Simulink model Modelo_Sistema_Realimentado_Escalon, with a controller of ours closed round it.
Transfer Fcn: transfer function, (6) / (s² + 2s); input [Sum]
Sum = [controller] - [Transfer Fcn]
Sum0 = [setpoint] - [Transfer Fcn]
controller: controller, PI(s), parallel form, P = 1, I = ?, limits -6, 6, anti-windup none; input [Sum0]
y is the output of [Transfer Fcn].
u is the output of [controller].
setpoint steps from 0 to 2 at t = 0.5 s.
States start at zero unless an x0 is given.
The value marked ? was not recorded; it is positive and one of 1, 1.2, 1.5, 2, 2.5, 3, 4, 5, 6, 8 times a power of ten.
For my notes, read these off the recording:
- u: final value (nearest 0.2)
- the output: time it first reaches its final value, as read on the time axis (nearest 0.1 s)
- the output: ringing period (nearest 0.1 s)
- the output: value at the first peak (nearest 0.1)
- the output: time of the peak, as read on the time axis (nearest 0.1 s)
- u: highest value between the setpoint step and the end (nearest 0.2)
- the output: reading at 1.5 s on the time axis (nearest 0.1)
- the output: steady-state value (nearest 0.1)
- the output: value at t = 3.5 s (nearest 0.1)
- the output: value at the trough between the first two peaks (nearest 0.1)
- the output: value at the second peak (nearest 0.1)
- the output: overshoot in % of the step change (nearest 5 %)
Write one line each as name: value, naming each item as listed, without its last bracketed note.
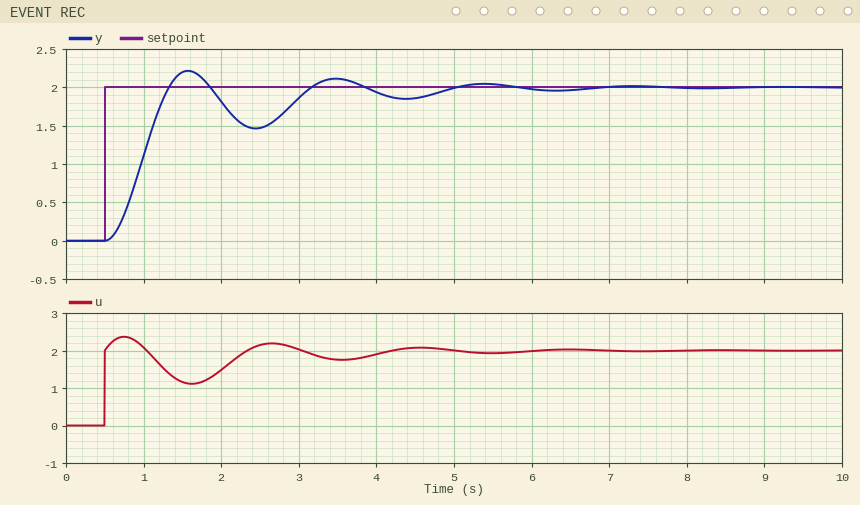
u: final value: 2.0
the output: time it first reaches its final value, as read on the time axis: 1.3 s
the output: ringing period: 1.9 s
the output: value at the first peak: 2.2
the output: time of the peak, as read on the time axis: 1.6 s
u: highest value between the setpoint step and the end: 2.4
the output: reading at 1.5 s on the time axis: 2.2
the output: steady-state value: 2.0
the output: value at t = 3.5 s: 2.1
the output: value at the trough between the first two peaks: 1.5
the output: value at the second peak: 2.1
the output: overshoot in % of the step change: 10 %
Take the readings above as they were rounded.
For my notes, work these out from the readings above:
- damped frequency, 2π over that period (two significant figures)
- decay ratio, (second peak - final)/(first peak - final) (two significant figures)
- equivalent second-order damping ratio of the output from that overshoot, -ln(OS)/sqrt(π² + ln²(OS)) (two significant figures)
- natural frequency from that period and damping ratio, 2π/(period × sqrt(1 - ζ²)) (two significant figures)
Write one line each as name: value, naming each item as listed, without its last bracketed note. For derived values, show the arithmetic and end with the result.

damped frequency, 2π over that period: 2π / 1.9 = 3.3 rad/s
decay ratio, (second peak - final)/(first peak - final): (2.1 - 2) / (2.2 - 2) = 0.50
equivalent second-order damping ratio of the output from that overshoot, -ln(OS)/sqrt(π² + ln²(OS)): ln(0.1) = -2.303; 2.303 / sqrt(9.870 + 5.302) = 0.59
natural frequency from that period and damping ratio, 2π/(period × sqrt(1 - ζ²)): 2π / (1.9 × sqrt(1 - 0.59²)) = 4.1 rad/s
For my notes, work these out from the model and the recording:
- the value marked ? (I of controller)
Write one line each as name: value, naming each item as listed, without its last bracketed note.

the value marked ?: 1.5
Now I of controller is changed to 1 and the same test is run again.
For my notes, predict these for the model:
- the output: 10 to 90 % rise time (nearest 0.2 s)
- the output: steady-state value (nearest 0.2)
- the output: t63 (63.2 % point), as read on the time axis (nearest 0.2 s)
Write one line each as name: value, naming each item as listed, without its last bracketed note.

the output: 10 to 90 % rise time: 0.6 s
the output: steady-state value: 2.0
the output: t63 (63.2 % point), as read on the time axis: 1.0 s
